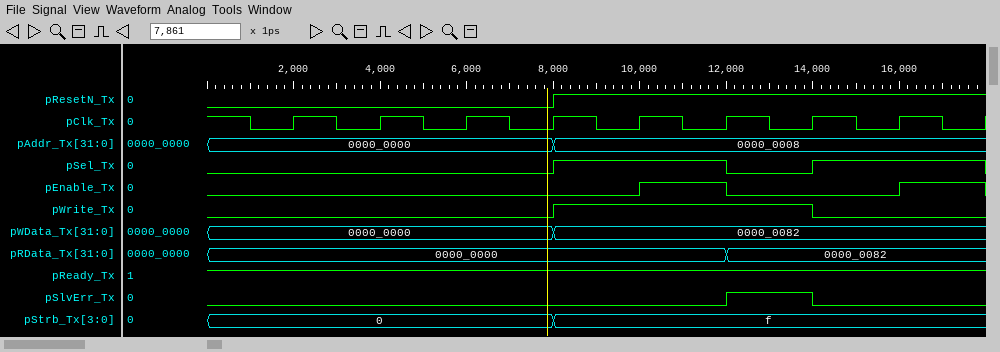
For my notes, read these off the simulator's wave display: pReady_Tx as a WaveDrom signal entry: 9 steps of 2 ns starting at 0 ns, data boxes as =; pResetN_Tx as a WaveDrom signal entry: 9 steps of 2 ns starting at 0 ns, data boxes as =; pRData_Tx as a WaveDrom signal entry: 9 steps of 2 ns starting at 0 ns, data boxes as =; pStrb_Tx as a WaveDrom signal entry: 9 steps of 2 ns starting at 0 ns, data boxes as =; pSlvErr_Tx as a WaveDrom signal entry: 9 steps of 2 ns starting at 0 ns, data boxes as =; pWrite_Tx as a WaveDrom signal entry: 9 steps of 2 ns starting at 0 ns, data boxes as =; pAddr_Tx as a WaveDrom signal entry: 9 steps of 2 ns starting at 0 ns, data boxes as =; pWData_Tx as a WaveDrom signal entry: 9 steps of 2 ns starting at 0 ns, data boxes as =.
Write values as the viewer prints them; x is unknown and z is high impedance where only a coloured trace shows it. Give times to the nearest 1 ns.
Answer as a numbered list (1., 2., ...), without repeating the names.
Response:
1. {name: 'pReady_Tx', wave: '1........'}
2. {name: 'pResetN_Tx', wave: '0...1....'}
3. {name: 'pRData_Tx', wave: '=.....=..', data: '0000_0000 0000_0082'}
4. {name: 'pStrb_Tx', wave: '=...=....', data: '0 f'}
5. {name: 'pSlvErr_Tx', wave: '0.....10.'}
6. {name: 'pWrite_Tx', wave: '0...1..0.'}
7. {name: 'pAddr_Tx', wave: '=...=....', data: '0000_0000 0000_0008'}
8. {name: 'pWData_Tx', wave: '=...=....', data: '0000_0000 0000_0082'}
